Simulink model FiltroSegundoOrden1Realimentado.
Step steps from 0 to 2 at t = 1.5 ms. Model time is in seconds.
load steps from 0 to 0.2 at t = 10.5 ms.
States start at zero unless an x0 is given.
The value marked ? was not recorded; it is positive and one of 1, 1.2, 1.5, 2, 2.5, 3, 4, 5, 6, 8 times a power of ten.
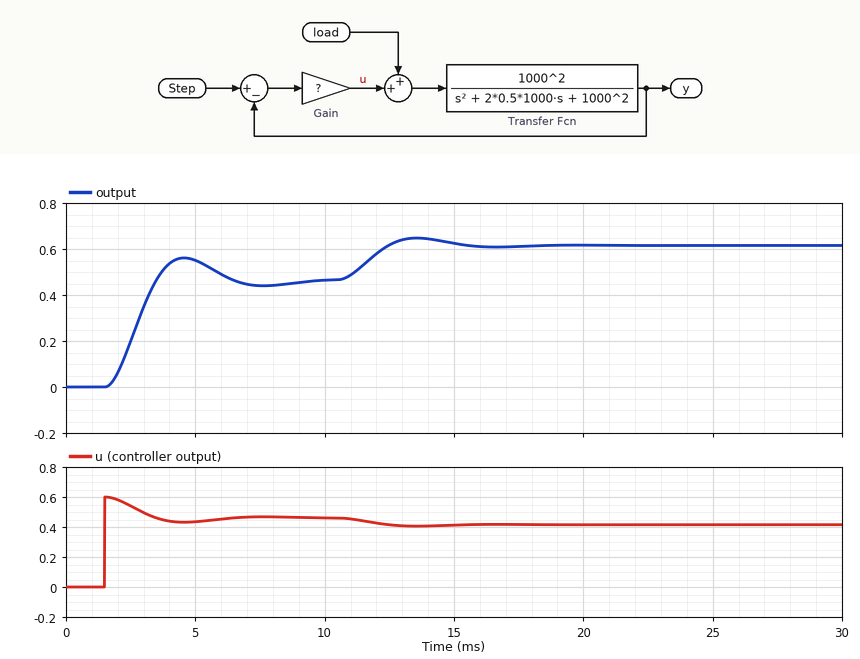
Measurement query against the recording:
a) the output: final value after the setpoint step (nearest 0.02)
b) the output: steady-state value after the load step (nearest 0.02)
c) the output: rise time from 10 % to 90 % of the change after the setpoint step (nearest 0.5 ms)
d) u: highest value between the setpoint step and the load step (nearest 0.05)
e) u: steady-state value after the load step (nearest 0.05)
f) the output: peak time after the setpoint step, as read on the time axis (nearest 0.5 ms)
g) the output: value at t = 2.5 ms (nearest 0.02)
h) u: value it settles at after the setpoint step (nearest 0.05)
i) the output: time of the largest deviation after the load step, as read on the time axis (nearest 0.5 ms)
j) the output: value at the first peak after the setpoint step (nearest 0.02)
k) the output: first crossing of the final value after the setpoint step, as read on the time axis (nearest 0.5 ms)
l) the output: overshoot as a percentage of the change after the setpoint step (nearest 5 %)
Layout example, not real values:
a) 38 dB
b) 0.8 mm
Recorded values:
a) 0.46
b) 0.62
c) 1.5 ms
d) 0.60
e) 0.40
f) 4.5 ms
g) 0.20
h) 0.45
i) 13.5 ms
j) 0.56
k) 3.5 ms
l) 20 %
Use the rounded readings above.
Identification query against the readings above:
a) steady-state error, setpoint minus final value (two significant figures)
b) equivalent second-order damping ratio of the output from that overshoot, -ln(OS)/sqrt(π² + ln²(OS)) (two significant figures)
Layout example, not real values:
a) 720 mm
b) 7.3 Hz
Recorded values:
a) 1.5
b) 0.46
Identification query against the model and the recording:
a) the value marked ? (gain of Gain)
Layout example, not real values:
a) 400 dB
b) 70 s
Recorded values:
a) 0.3
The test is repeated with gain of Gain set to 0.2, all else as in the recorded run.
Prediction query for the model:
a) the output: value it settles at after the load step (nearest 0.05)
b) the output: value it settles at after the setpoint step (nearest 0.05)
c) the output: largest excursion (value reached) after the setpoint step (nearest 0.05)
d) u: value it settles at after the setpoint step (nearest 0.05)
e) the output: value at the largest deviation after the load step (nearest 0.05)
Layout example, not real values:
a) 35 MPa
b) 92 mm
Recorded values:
a) 0.50
b) 0.35
c) 0.40
d) 0.35
e) 0.55
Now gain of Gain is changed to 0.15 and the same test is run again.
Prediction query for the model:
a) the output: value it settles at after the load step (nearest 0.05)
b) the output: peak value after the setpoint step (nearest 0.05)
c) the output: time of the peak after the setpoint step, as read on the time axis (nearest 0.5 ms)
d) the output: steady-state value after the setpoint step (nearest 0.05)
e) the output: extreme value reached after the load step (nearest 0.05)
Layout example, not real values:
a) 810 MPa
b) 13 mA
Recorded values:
a) 0.45
b) 0.30
c) 5.0 ms
d) 0.25
e) 0.45
